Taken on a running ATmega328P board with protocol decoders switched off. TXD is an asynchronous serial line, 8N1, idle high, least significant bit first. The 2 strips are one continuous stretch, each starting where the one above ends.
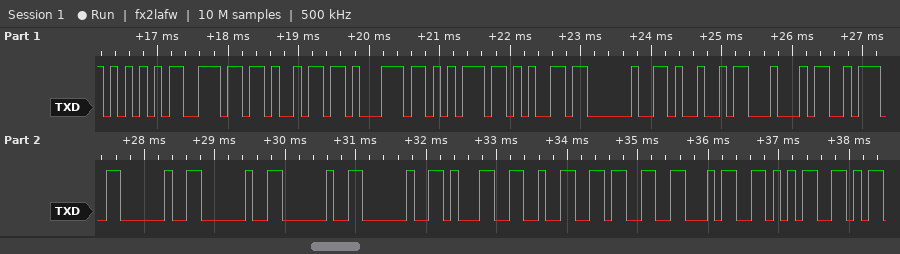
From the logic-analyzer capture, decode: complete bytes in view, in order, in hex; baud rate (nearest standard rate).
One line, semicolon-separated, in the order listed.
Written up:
55 6E 69 71 75 65 20 49 44 3A 20 20 20 20 31 32 33 34 35; 9600 baud
